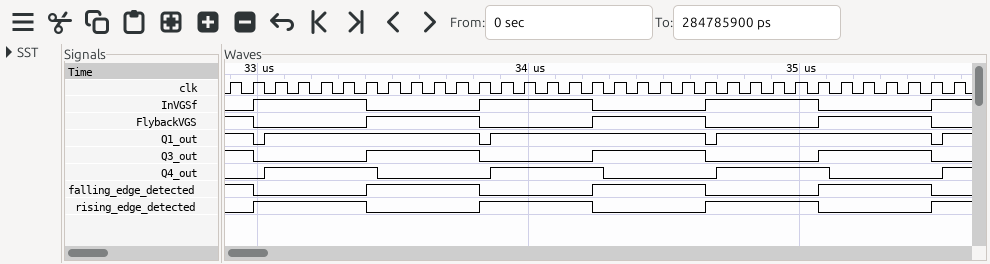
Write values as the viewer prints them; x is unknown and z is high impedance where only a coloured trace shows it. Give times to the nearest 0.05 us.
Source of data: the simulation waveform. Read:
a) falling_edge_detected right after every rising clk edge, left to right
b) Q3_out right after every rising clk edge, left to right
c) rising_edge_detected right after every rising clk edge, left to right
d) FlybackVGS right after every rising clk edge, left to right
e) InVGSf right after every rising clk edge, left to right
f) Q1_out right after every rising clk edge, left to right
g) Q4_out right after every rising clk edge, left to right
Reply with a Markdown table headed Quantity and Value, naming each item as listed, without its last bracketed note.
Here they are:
| Quantity | Value |
|---|---|
| falling_edge_detected right after every rising clk edge, left to right | 1 0 0 0 0 0 1 1 1 1 1 0 0 0 0 0 1 1 1 1 1 0 0 0 0 0 1 1 1 1 1 0 0 |
| Q3_out right after every rising clk edge, left to right | 1 0 0 0 0 0 1 1 1 1 1 0 0 0 0 0 1 1 1 1 1 0 0 0 0 0 1 1 1 1 1 0 0 |
| rising_edge_detected right after every rising clk edge, left to right | 0 1 1 1 1 1 0 0 0 0 0 1 1 1 1 1 0 0 0 0 0 1 1 1 1 1 0 0 0 0 0 1 1 |
| FlybackVGS right after every rising clk edge, left to right | 1 0 0 0 0 0 1 1 1 1 1 0 0 0 0 0 1 1 1 1 1 0 0 0 0 0 1 1 1 1 1 0 0 |
| InVGSf right after every rising clk edge, left to right | 0 1 1 1 1 1 0 0 0 0 0 1 1 1 1 1 0 0 0 0 0 1 1 1 1 1 0 0 0 0 0 1 1 |
| Q1_out right after every rising clk edge, left to right | 1 0 1 1 1 1 1 1 1 1 1 0 1 1 1 1 1 1 1 1 1 0 1 1 1 1 1 1 1 1 1 0 1 |
| Q4_out right after every rising clk edge, left to right | 0 0 1 1 1 1 1 0 0 0 0 0 1 1 1 1 1 0 0 0 0 0 1 1 1 1 1 0 0 0 0 0 1 |
